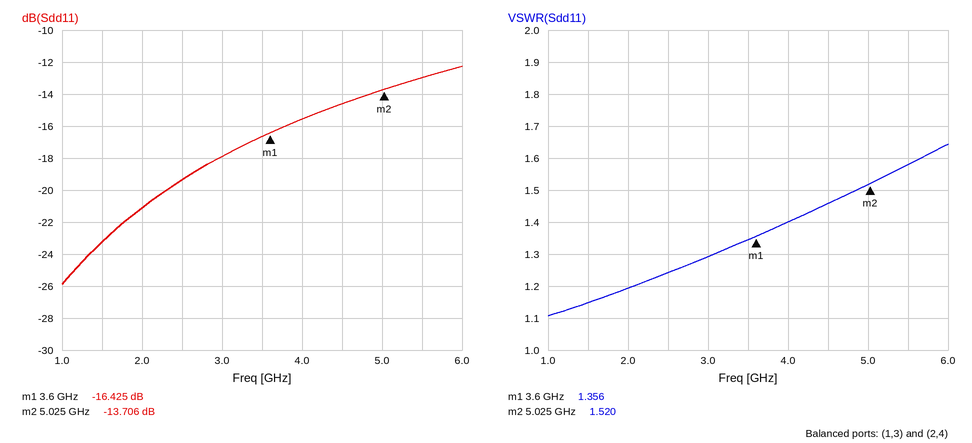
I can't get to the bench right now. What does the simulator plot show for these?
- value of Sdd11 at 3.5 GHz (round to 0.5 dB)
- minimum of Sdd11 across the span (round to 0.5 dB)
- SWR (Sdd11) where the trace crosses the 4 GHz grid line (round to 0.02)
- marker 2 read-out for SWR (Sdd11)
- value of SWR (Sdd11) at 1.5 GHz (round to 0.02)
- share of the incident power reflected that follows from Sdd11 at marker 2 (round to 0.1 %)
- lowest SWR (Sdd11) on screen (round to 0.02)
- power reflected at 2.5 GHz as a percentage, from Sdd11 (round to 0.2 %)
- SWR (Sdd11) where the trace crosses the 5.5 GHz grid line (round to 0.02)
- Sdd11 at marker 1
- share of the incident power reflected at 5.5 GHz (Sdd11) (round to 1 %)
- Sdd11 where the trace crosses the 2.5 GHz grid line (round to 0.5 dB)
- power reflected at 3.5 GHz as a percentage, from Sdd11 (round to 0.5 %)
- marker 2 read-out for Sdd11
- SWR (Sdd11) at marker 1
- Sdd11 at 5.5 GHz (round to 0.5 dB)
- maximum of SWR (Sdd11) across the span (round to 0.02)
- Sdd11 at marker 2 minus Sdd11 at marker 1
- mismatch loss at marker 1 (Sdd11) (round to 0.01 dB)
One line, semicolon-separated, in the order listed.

-16.5 dB; -26.0 dB; 1.40; 1.520; 1.14; 4.3 %; 1.10; 1.2 %; 1.58; -16.425 dB; 5 %; -19.5 dB; 2.0 %; -13.706 dB; 1.356; -13.0 dB; 1.64; 2.719 dB; 0.10 dB
